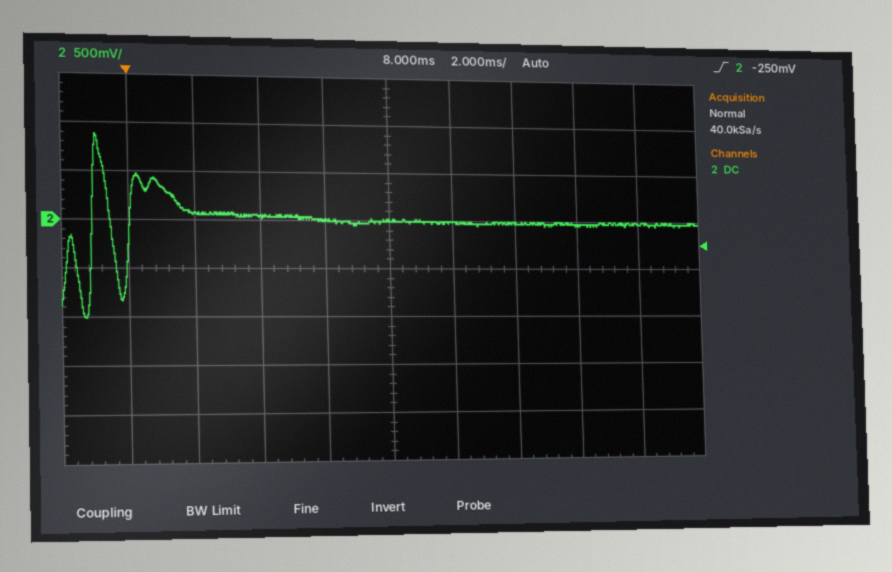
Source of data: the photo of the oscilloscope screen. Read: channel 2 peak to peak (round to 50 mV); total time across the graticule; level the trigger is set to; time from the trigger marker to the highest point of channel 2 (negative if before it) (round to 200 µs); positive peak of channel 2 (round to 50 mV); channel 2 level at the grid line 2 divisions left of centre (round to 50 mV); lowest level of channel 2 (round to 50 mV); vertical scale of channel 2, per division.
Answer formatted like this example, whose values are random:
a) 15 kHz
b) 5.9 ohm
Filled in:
a) 1.90 V
b) 20 ms
c) -250 mV
d) -1.0 ms
e) 900 mV
f) 50 mV
g) -1.00 V
h) 500 mV
